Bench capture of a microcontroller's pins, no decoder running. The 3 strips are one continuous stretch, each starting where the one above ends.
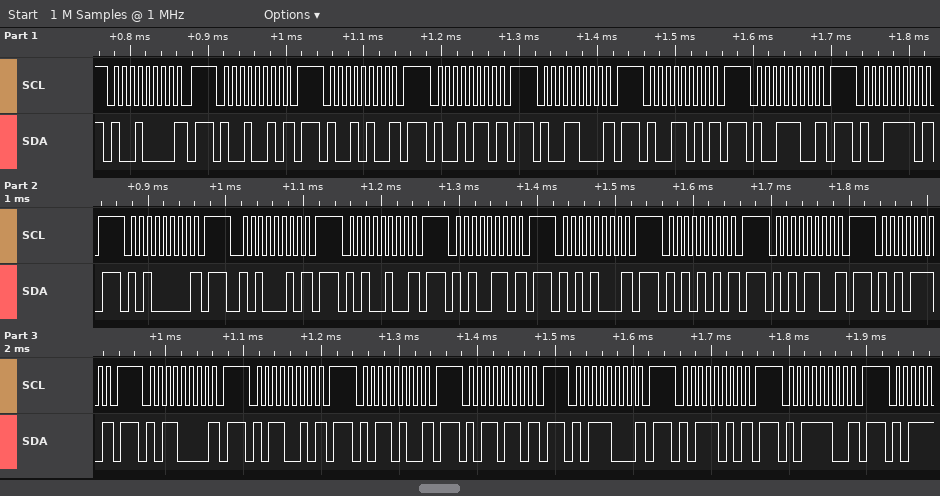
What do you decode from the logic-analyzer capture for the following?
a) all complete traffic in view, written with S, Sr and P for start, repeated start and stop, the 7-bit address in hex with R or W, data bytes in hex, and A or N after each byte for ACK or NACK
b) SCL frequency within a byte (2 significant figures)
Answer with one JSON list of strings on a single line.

["S 48W N P S 49W N P S 4AW N P S 4BW N P S 4CW N P S 4DW N P S 4EW N P S 4FW N P S 50W N P S 51W N P S 52W N P S 53W N P S 54W N P S 55W N P S 56W N P S 57W N P S 58W N P S 59W N P S 5AW N P S 5BW N P S 5CW N P S 5DW N P S 5EW N P", "100 kHz"]
